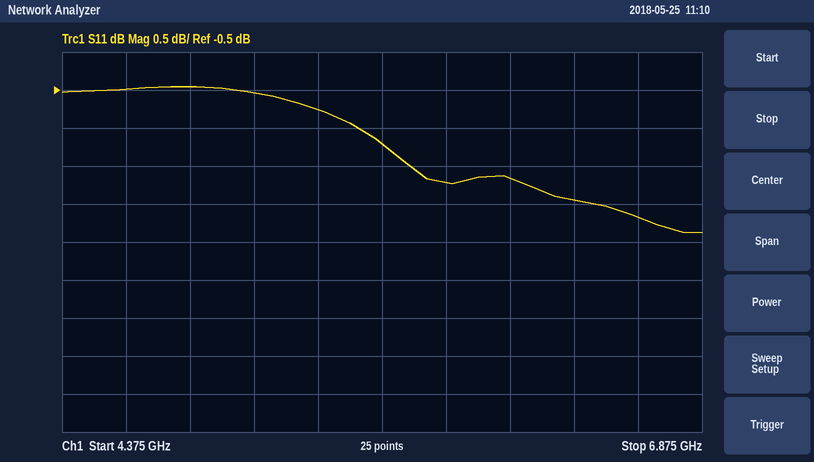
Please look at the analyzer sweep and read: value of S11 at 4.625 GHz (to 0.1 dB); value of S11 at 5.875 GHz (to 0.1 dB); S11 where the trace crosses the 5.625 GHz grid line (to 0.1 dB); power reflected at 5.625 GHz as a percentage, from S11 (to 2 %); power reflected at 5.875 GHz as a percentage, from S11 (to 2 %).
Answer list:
-0.5 dB
-1.7 dB
-1.2 dB
76 %
68 %
